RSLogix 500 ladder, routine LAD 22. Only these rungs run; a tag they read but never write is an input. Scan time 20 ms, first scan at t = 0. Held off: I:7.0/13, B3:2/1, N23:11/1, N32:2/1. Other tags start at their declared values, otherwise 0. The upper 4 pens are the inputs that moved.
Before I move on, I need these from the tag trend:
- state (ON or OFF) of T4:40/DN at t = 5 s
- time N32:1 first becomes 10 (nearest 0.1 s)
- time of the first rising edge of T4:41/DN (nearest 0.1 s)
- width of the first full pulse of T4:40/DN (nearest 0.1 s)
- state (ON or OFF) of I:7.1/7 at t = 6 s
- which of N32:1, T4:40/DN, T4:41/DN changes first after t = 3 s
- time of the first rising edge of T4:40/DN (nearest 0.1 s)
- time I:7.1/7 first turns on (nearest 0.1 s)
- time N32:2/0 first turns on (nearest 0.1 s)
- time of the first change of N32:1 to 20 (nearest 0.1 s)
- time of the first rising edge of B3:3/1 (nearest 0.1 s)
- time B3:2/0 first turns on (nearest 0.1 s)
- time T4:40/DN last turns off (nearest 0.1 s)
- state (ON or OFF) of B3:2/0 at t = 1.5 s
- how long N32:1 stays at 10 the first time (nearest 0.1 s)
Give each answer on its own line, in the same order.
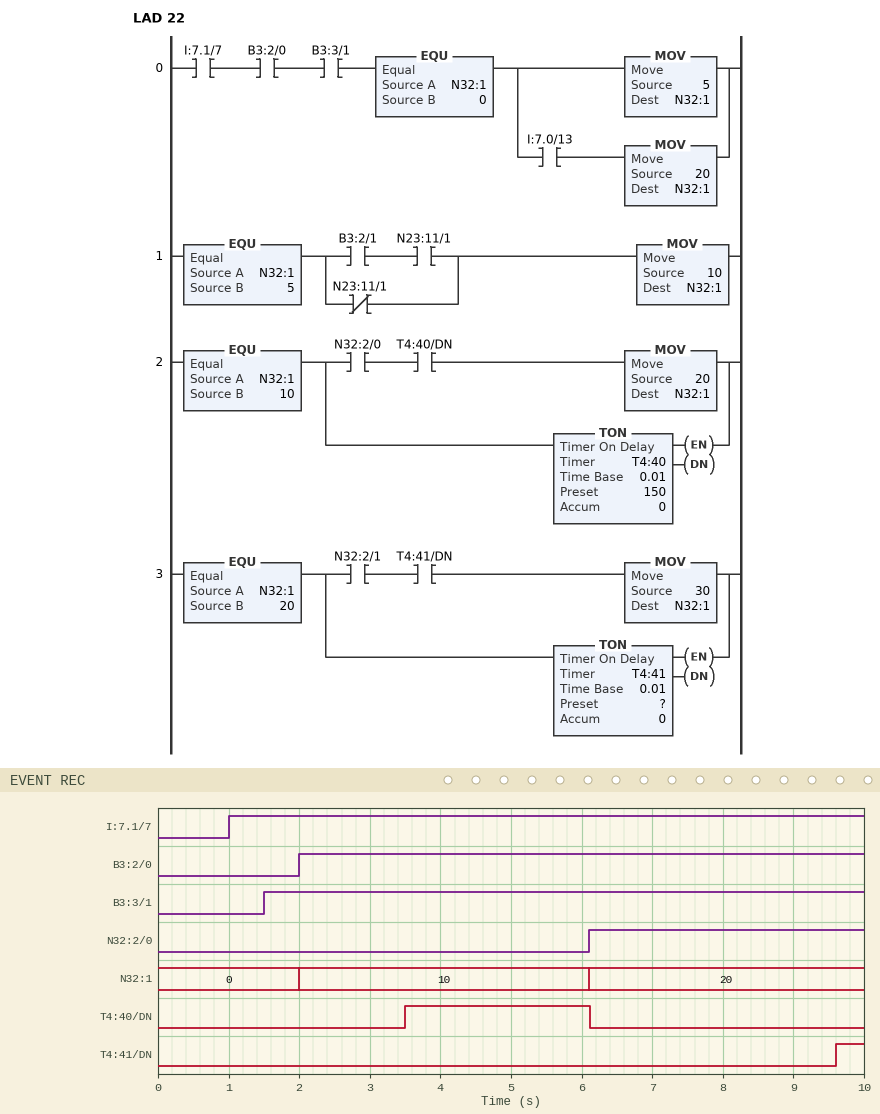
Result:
ON
2.0 s
9.6 s
2.6 s
ON
T4:40/DN
3.5 s
1.0 s
6.1 s
6.1 s
1.5 s
2.0 s
6.1 s
OFF
4.1 s
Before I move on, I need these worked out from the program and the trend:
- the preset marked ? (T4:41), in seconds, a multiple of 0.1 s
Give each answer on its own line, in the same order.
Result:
3.5 s
